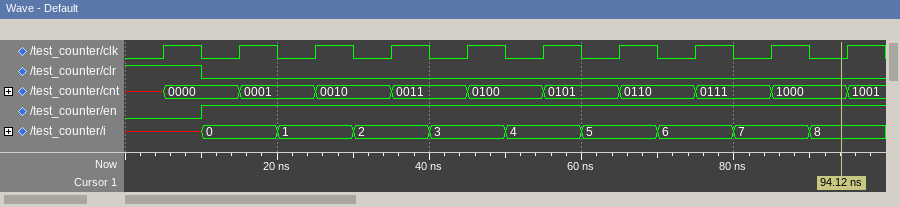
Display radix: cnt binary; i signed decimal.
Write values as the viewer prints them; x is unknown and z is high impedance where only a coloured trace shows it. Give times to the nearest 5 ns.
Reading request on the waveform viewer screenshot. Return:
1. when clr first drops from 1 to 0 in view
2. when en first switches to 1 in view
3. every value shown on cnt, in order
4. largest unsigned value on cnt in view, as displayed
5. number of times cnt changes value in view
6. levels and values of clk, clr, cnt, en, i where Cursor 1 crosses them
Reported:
10 ns
10 ns
x, 0000, 0001, 0010, 0011, 0100, 0101, 0110, 0111, 1000, 1001
1001
10
clk=0, clr=0, cnt=1000, en=1, i=8
